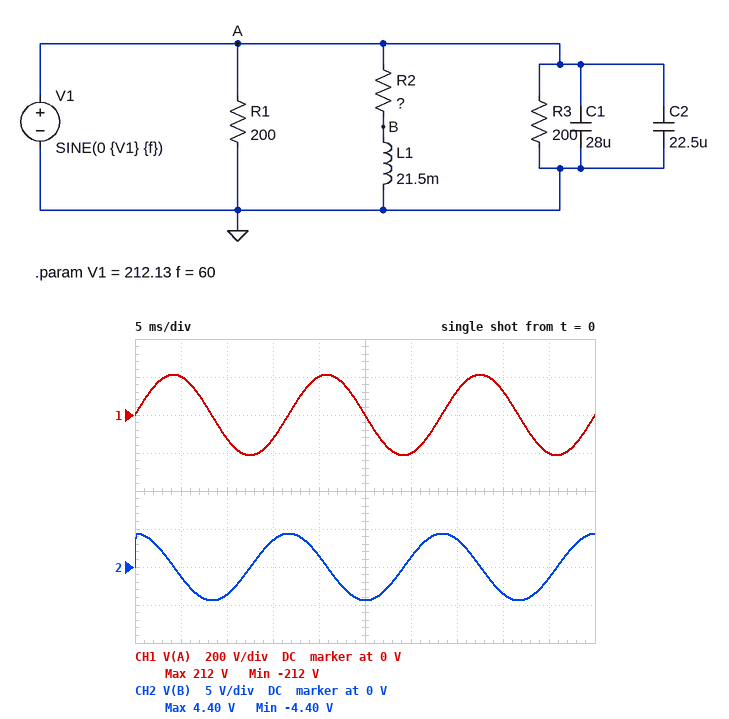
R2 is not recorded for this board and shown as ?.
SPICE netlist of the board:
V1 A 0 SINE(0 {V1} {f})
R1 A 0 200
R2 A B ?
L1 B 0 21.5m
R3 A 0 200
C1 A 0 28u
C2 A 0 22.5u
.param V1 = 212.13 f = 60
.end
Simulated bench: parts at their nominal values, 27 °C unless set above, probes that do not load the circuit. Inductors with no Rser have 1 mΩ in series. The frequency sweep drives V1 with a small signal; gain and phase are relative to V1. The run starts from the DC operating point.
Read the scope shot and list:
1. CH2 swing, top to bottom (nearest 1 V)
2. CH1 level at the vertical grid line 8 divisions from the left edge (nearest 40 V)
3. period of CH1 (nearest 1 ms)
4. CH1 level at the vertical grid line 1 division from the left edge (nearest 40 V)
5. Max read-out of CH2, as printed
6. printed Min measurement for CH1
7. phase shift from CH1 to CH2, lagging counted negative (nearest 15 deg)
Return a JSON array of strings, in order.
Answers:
["9 V", "120 V", "17 ms", "200 V", "4.40 V", "-212 V", "90 deg"]
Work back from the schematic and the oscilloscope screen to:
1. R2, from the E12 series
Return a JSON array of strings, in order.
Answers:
["390 Ω"]
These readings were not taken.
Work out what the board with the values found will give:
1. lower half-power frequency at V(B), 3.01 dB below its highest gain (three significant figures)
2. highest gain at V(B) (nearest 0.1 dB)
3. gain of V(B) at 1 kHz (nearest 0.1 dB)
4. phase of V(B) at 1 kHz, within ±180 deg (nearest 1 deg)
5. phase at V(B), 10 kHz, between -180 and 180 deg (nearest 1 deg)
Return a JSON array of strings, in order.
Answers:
["2.89 kHz", "0 dB", "-9.7 dB", "71 deg", "16 deg"]
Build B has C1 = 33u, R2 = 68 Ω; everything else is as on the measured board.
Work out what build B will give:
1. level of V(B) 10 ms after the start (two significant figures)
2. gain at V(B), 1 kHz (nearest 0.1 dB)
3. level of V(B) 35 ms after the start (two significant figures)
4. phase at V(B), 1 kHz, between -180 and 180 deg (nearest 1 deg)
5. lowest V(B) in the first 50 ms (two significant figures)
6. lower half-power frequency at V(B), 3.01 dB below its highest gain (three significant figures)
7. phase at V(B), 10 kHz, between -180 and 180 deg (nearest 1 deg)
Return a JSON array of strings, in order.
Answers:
["-22 V", "-1.0 dB", "22 V", "27 deg", "-25 V", "503 Hz", "3 deg"]
